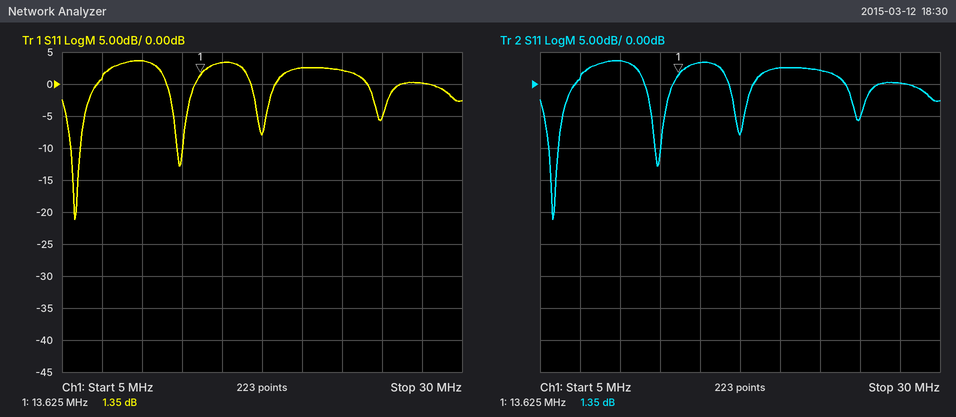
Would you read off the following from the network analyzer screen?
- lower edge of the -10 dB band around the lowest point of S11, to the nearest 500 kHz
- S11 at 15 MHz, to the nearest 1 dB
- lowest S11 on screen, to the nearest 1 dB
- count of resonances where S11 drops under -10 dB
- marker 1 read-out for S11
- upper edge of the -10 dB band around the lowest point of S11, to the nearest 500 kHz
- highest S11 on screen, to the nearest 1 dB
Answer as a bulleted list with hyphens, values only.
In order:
- 5.5 MHz
- 3 dB
- -21 dB
- 2
- 1.35 dB
- 6.0 MHz
- 4 dB
